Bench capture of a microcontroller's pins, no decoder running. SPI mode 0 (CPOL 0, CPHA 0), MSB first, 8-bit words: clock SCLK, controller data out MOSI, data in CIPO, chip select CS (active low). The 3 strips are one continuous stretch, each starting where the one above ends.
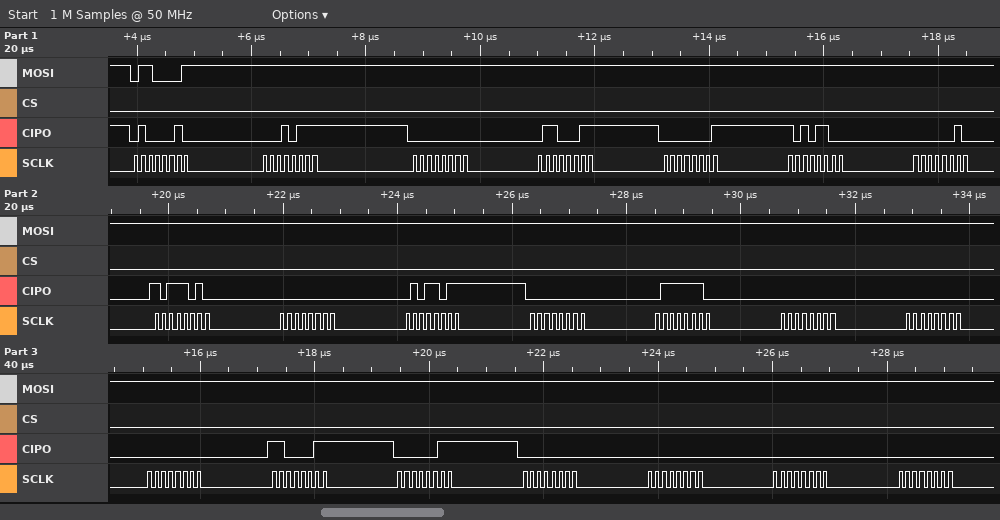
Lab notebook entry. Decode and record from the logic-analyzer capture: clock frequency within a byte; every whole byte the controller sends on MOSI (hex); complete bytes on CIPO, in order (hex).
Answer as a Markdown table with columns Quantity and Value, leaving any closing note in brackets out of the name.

| Quantity | Value |
|---|---|
| clock frequency within a byte | 8 MHz |
| every whole byte the controller sends on MOSI | 61 FF FF FF FF FF FF FF FF FF FF FF FF FF FF FF FF FF FF FF FF |
| complete bytes on CIPO, in order | 42 17 00 63 01 AC 02 BA 00 5B 00 7E 00 00 00 C3 03 00 00 00 00 |
